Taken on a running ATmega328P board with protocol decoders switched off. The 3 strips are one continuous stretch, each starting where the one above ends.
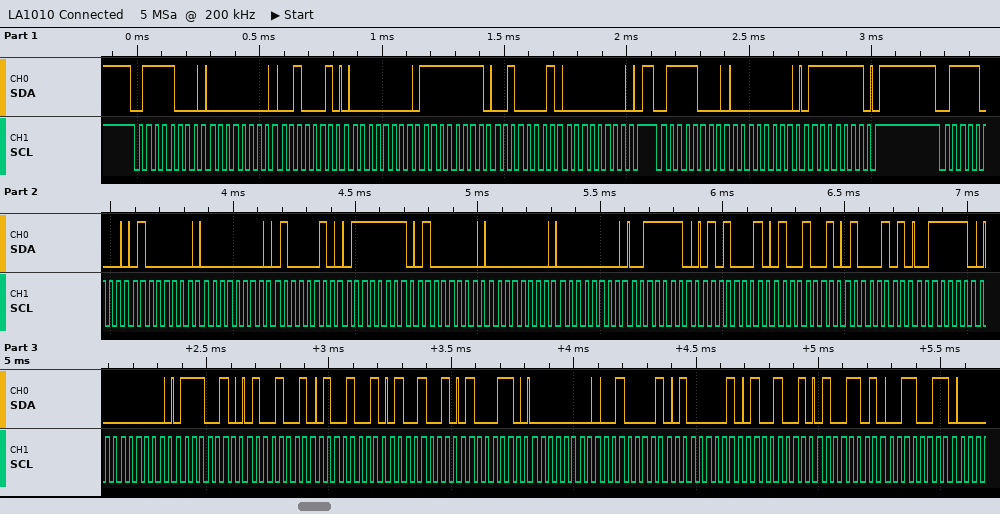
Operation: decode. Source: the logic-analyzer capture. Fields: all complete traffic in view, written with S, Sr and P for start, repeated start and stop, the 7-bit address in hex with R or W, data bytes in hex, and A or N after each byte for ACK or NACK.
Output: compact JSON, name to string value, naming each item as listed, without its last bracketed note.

{"all complete traffic in view, written with S, Sr and P for start, repeated start and stop, the 7-bit address in hex with R or W, data bytes in hex, and A or N after each byte for ACK or NACK": "S 3CW A 00 A 22 A 00 A FF A 21 A 00 A P S 3CW A 00 A 7F A P S 3CW A 40 A 00 A 42 A 7F A 40 A 00 A 00 A 3E A 51 A 49 A 45 A 3E A 00 A 72 A 49 A 49 A 49 A 46 A 00 A 21 A 41 A 49 A 4D A 33 A"}
